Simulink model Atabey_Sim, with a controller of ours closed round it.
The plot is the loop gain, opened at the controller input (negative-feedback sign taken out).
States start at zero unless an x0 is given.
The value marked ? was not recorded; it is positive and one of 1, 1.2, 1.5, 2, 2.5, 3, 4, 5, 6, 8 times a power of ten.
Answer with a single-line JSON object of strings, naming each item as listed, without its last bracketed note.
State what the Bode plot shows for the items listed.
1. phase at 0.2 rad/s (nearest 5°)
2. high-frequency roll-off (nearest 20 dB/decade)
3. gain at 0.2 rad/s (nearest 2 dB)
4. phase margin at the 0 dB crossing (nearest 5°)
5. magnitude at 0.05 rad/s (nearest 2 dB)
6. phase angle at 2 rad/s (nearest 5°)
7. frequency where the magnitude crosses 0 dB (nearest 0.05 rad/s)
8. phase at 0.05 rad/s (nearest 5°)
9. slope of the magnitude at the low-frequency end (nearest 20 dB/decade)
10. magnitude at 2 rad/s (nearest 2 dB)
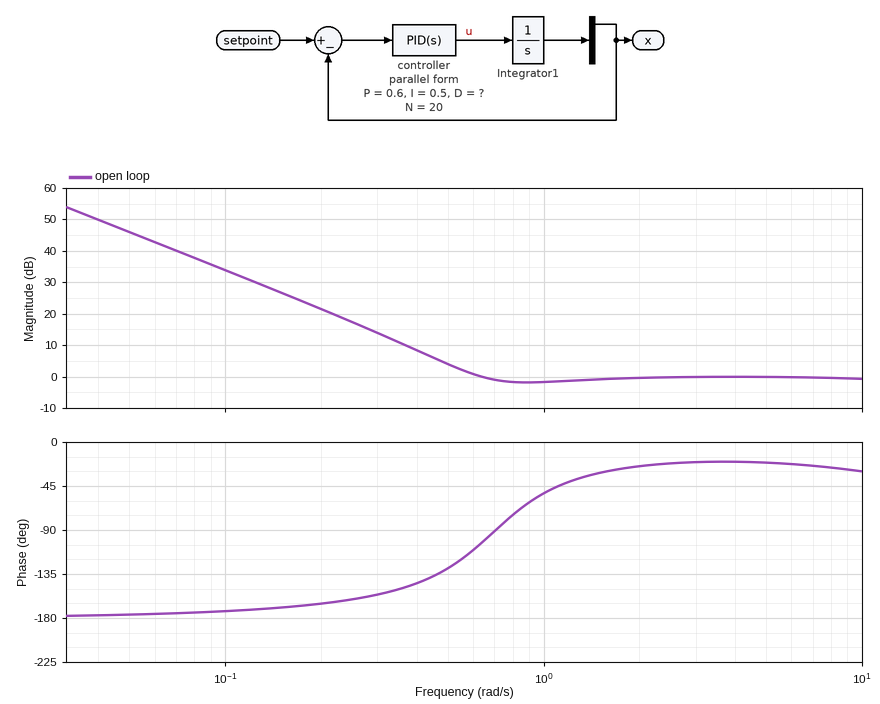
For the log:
{"phase at 0.2 rad/s": "-165°", "high-frequency roll-off": "0 dB/decade", "gain at 0.2 rad/s": "22 dB", "phase margin at the 0 dB crossing": "75°", "magnitude at 0.05 rad/s": "46 dB", "phase angle at 2 rad/s": "-25°", "frequency where the magnitude crosses 0 dB": "0.65 rad/s", "phase at 0.05 rad/s": "-175°", "slope of the magnitude at the low-frequency end": "-40 dB/decade", "magnitude at 2 rad/s": "0 dB"}
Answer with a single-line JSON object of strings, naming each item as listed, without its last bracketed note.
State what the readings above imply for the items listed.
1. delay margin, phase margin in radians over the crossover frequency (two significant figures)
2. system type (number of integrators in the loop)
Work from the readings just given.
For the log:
{"delay margin, phase margin in radians over the crossover frequency": "2.0 s", "system type": "2"}
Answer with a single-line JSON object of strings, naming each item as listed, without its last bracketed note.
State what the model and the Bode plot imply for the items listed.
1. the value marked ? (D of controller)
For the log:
{"the value marked ?": "1"}
